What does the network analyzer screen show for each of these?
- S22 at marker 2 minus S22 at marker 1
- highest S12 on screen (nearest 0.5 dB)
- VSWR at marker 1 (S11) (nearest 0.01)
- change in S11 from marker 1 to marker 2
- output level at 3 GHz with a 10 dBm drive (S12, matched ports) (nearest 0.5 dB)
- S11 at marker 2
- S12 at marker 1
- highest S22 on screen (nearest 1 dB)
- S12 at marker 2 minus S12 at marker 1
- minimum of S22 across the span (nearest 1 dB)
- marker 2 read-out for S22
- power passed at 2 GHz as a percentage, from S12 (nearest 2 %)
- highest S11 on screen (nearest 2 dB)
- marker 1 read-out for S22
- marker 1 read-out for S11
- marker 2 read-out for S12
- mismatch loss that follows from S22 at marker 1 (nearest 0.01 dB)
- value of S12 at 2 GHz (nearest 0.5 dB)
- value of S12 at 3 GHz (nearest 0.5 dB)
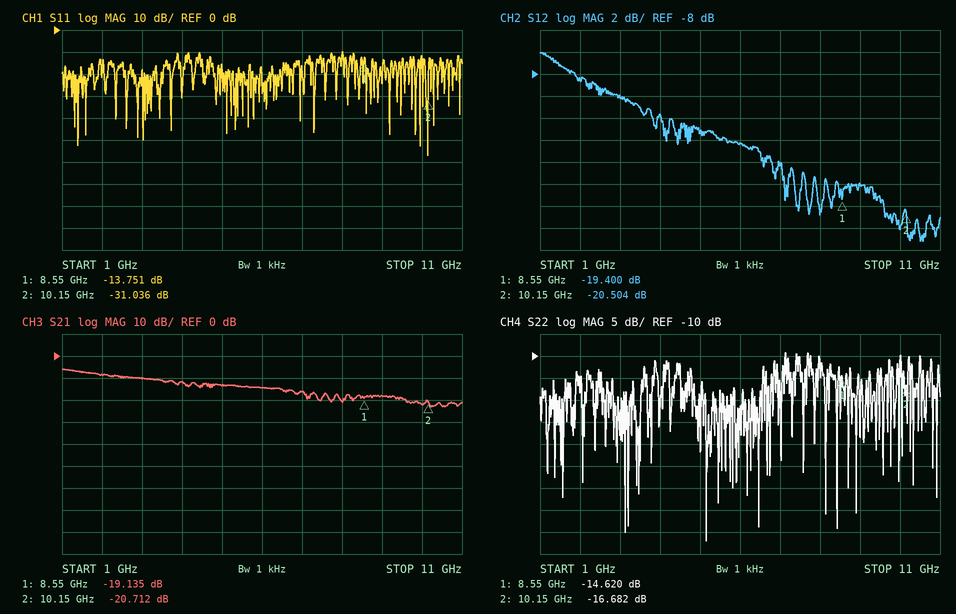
-2.062 dB
-6.0 dB
1.52
-17.285 dB
0.0 dBm
-31.036 dB
-19.400 dB
-9 dB
-1.104 dB
-52 dB
-16.682 dB
14 %
-10 dB
-14.620 dB
-13.751 dB
-20.504 dB
0.15 dB
-8.5 dB
-10.0 dB
